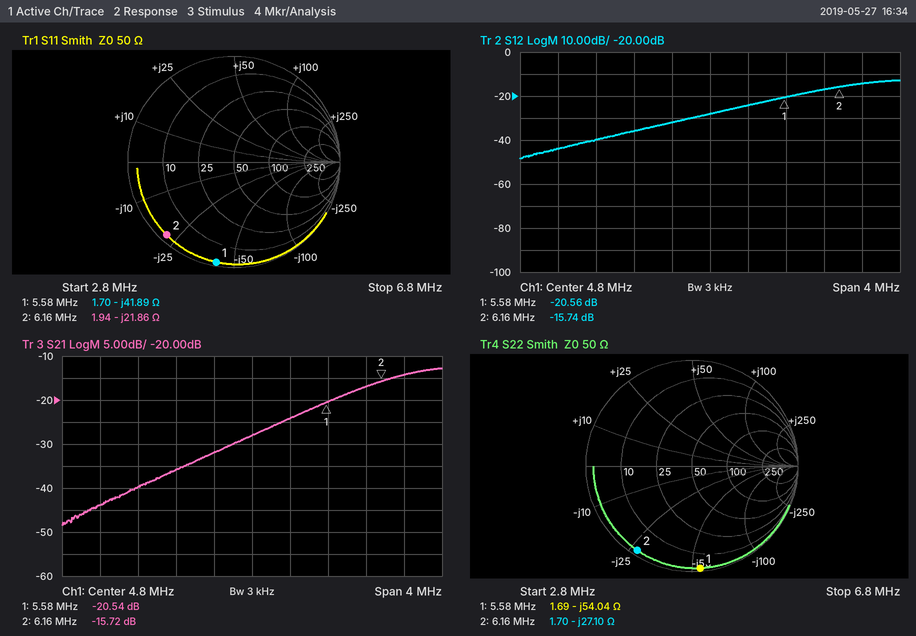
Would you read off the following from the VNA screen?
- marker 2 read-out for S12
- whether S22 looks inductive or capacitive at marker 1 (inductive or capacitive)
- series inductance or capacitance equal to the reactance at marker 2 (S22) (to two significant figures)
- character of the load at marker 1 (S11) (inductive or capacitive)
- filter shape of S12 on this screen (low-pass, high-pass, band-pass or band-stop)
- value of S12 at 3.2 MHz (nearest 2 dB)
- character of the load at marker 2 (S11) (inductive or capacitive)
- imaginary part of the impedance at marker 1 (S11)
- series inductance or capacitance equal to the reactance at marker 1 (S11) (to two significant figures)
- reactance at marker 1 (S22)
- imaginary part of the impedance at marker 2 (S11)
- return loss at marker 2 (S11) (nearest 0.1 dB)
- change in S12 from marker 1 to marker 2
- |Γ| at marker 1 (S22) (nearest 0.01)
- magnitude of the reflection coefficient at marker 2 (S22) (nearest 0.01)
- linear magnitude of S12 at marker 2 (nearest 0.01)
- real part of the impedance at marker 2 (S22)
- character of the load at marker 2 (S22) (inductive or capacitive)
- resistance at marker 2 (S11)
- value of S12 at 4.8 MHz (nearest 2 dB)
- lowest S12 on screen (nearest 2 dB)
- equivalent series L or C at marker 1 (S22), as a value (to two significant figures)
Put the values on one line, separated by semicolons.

-15.74 dB; capacitive; 950 pF; capacitive; high-pass; -44 dB; capacitive; -41.89 Ω; 680 pF; -54.04 Ω; -21.86 Ω; 0.6 dB; 4.82 dB; 0.97; 0.95; 0.16; 1.70 Ω; capacitive; 1.94 Ω; -28 dB; -48 dB; 530 pF
